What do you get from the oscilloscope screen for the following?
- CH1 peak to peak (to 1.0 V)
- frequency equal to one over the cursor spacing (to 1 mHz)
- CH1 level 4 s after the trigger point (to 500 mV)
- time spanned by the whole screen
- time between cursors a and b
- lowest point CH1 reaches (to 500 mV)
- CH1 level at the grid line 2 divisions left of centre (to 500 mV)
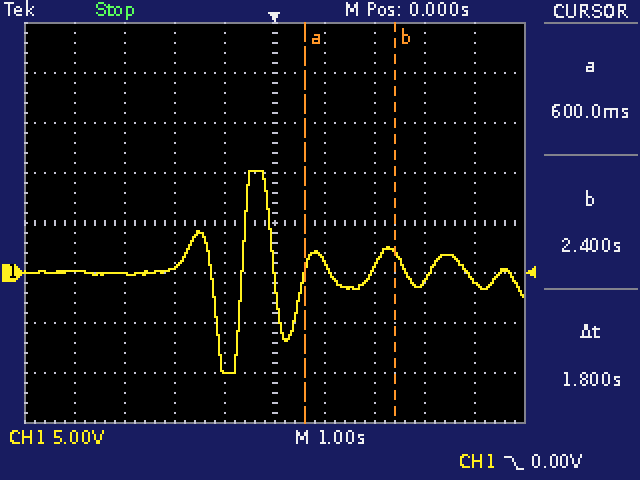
20.0 V
556 mHz
-1.0 V
10 s
1.8 s
-10.0 V
500 mV
